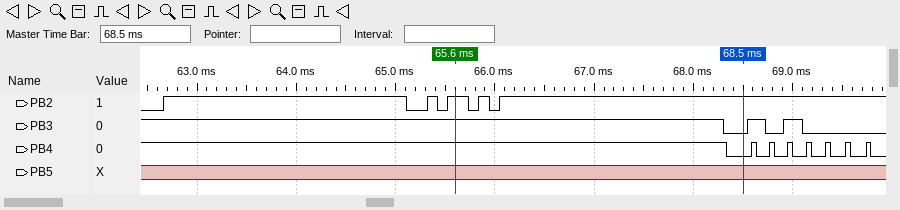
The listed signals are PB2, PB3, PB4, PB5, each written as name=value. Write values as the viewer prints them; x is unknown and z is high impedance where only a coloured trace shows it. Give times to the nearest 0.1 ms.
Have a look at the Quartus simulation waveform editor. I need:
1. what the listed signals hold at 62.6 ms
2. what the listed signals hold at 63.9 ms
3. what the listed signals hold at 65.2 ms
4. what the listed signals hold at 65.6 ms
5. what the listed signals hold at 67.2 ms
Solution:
PB2=0, PB3=1, PB4=1, PB5=x
PB2=1, PB3=1, PB4=1, PB5=x
PB2=0, PB3=1, PB4=1, PB5=x
PB2=1, PB3=1, PB4=1, PB5=x
PB2=1, PB3=1, PB4=1, PB5=x
